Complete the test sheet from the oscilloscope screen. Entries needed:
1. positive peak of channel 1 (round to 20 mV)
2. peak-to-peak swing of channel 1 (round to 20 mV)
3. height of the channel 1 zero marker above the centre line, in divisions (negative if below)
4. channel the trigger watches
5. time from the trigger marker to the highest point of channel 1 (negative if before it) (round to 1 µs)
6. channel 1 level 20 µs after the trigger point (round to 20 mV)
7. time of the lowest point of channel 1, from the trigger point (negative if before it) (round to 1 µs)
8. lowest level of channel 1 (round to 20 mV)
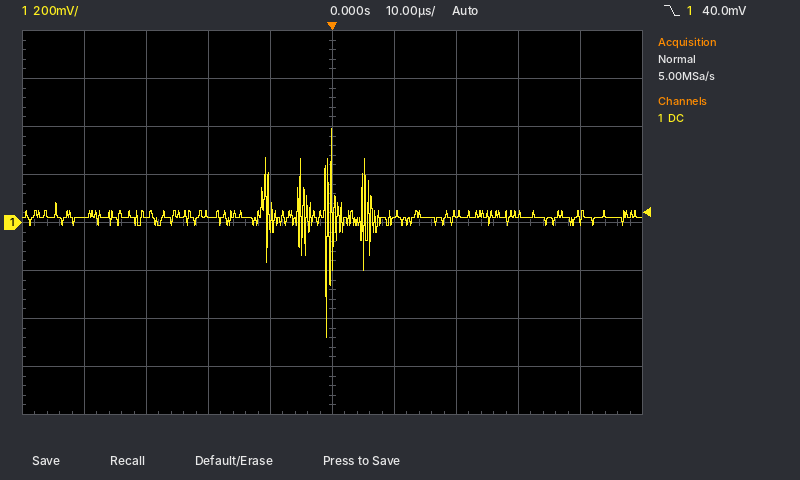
400 mV
880 mV
0.0 div
channel 1
0 µs
40 mV
-1 µs
-480 mV
